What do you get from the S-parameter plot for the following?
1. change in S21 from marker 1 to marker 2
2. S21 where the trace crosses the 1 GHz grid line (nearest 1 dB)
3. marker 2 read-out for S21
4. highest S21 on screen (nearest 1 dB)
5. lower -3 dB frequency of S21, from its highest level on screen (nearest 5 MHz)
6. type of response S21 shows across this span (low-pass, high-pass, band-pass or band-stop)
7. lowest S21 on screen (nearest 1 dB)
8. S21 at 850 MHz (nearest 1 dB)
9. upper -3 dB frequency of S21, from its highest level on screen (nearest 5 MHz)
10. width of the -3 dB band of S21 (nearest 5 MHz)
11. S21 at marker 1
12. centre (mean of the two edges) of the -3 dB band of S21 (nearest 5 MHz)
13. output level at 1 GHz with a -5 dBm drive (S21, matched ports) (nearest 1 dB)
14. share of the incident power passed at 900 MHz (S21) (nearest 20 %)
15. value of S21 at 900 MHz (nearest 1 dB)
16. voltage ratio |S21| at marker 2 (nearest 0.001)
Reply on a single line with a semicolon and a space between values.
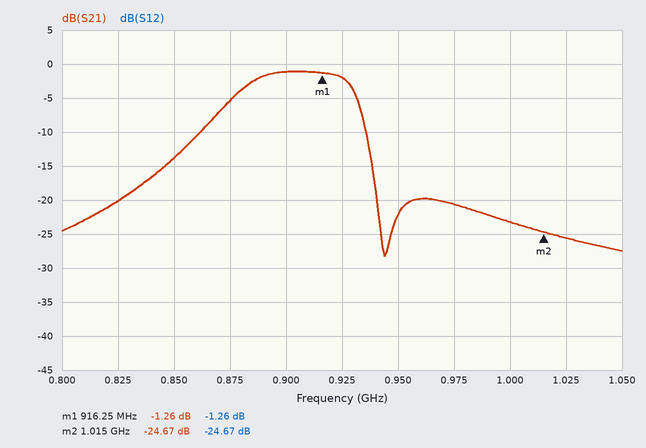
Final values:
-23.41 dB; -23 dB; -24.67 dB; -1 dB; 880 MHz; band-pass; -28 dB; -14 dB; 930 MHz; 50 MHz; -1.26 dB; 905 MHz; -28 dBm; 80 %; -1 dB; 0.058
